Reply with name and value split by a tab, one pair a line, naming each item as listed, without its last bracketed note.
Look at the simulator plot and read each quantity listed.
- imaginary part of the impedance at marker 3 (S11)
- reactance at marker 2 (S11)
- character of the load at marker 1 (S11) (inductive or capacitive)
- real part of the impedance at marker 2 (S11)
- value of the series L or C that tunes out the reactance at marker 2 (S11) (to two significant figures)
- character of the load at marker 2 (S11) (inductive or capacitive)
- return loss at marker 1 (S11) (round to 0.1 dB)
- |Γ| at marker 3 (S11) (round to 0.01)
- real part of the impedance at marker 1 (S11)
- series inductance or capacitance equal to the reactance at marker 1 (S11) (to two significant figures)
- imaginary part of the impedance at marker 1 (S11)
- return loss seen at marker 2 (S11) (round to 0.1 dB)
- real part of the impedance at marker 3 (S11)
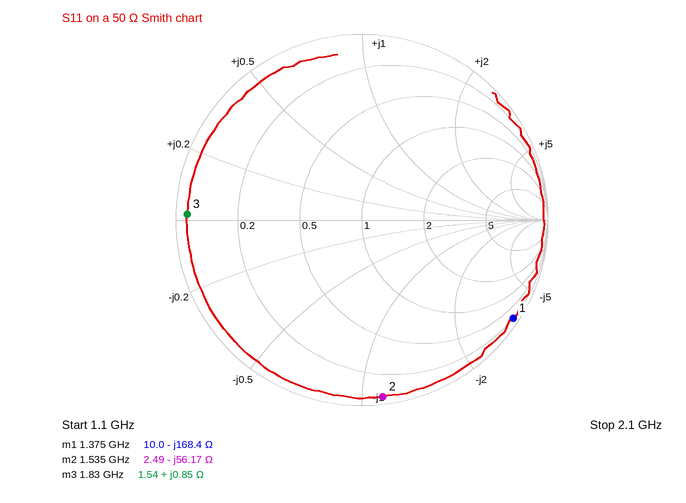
imaginary part of the impedance at marker 3	+0.85 Ω
reactance at marker 2	-56.17 Ω
character of the load at marker 1 (S11)	capacitive
real part of the impedance at marker 2	2.49 Ω
value of the series L or C that tunes out the reactance at marker 2 (S11)	5.8 nH
character of the load at marker 2 (S11)	capacitive
return loss at marker 1 (S11)	0.3 dB
|Γ| at marker 3 (S11)	0.94
real part of the impedance at marker 1	10.0 Ω
series inductance or capacitance equal to the reactance at marker 1 (S11)	690 fF
imaginary part of the impedance at marker 1	-168.4 Ω
return loss seen at marker 2 (S11)	0.4 dB
real part of the impedance at marker 3	1.54 Ω
